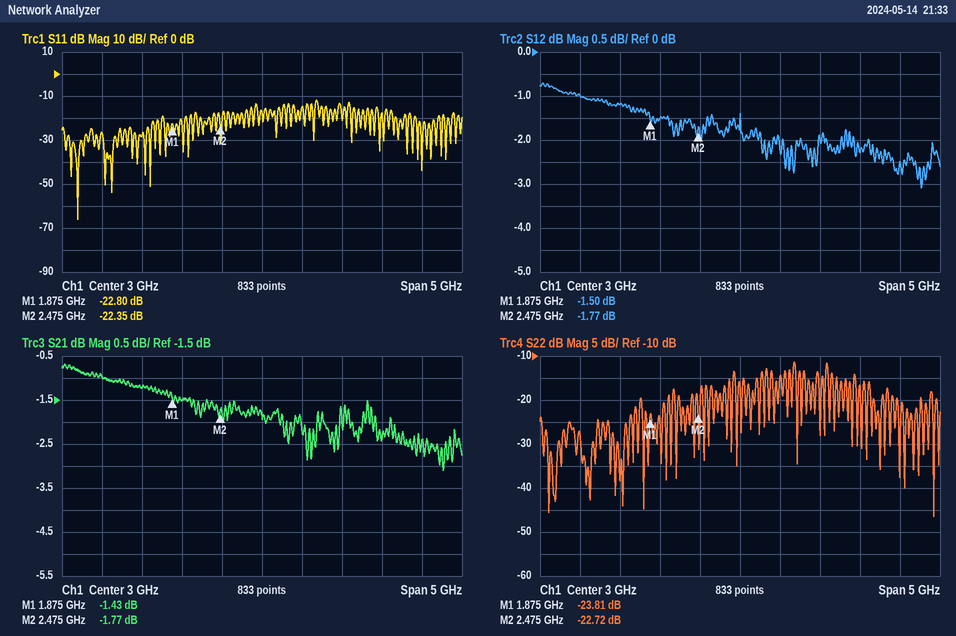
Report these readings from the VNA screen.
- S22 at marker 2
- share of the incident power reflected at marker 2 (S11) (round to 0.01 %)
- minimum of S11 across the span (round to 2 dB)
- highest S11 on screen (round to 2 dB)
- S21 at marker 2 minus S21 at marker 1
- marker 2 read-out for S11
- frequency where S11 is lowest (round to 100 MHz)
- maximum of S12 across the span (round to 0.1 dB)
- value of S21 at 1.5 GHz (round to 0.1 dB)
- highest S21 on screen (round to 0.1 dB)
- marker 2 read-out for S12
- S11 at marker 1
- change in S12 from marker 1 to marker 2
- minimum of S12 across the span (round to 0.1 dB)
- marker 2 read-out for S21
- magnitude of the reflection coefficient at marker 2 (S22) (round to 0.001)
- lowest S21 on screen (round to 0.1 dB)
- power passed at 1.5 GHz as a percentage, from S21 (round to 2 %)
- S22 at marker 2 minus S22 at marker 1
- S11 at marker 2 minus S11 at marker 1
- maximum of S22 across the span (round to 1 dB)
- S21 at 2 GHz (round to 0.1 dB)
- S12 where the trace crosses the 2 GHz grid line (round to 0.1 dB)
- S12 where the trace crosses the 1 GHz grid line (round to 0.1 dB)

-22.72 dB
0.58 %
-66 dB
-12 dB
-0.34 dB
-22.35 dB
700 MHz
-0.7 dB
-1.2 dB
-0.7 dB
-1.77 dB
-22.80 dB
-0.27 dB
-3.1 dB
-1.77 dB
0.073
-3.1 dB
76 %
1.09 dB
0.45 dB
-11 dB
-1.5 dB
-1.5 dB
-1.0 dB
